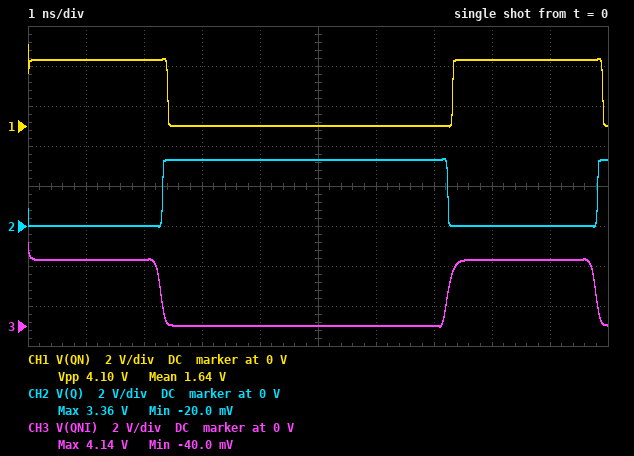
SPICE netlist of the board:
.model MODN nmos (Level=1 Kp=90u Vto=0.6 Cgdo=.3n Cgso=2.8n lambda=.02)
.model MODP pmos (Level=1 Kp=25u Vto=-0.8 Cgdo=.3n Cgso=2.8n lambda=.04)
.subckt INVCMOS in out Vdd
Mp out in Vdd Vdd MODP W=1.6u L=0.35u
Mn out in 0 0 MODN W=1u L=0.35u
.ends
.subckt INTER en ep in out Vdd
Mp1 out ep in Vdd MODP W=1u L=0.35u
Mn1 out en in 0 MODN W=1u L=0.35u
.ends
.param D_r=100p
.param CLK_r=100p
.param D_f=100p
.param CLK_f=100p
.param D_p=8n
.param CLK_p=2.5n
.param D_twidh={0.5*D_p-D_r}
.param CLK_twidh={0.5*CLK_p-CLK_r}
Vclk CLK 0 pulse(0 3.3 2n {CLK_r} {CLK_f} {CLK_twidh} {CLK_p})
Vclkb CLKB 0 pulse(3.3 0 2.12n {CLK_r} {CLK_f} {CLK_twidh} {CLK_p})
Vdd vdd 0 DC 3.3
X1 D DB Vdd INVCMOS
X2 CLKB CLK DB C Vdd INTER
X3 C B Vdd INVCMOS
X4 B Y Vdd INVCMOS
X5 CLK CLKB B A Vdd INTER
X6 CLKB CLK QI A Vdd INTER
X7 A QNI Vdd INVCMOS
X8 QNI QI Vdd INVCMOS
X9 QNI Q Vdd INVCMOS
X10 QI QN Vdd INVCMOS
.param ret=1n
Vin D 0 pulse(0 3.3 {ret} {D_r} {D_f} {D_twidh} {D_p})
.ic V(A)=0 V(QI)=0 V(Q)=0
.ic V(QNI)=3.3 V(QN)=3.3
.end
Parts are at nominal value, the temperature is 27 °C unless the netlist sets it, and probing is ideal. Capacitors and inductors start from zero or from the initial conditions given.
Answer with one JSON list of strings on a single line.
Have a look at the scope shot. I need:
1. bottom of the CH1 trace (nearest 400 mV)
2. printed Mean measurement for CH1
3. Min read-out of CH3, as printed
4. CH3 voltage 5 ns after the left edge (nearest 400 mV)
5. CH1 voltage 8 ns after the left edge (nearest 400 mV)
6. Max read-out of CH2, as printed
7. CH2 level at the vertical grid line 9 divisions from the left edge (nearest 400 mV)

["0 V", "1.64 V", "-40.0 mV", "0 V", "3.2 V", "3.36 V", "0 V"]
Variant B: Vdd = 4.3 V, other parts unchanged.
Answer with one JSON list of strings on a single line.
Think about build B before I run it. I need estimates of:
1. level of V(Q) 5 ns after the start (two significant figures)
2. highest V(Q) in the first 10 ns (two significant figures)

["4.3 V", "4.4 V"]
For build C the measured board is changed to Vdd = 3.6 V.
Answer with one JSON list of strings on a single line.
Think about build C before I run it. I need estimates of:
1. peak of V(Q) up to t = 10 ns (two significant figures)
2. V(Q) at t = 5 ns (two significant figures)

["3.7 V", "3.6 V"]
